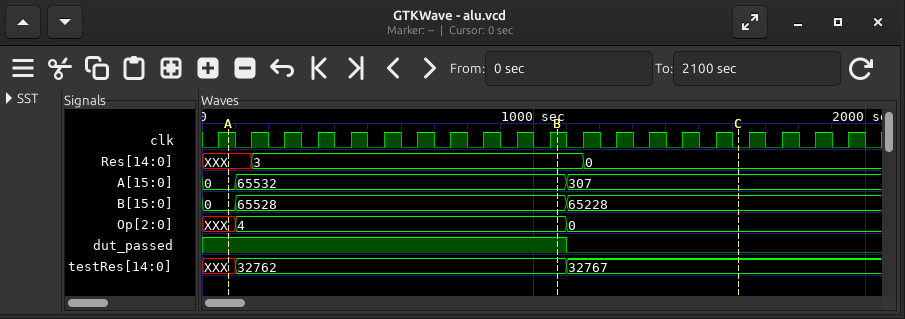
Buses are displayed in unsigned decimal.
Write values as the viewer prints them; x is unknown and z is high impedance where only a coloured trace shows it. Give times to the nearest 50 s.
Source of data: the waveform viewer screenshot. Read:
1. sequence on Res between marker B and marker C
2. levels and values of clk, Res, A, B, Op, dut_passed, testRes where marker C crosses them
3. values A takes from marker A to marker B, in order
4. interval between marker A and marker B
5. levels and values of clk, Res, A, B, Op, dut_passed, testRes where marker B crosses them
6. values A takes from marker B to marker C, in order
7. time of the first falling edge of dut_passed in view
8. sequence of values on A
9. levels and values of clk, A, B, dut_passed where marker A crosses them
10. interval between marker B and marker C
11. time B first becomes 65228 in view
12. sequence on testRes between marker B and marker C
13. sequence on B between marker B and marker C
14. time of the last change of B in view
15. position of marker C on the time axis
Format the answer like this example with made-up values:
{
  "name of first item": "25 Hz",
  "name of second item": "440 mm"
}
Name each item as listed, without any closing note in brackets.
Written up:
{
  "sequence on Res between marker B and marker C": "3, 0",
  "levels and values of clk, Res, A, B, Op, dut_passed, testRes where marker C crosses them": "clk=0, Res=0, A=307, B=65228, Op=0, dut_passed=0, testRes=32767",
  "values A takes from marker A to marker B, in order": "0, 65532",
  "interval between marker A and marker B": "1000 s",
  "levels and values of clk, Res, A, B, Op, dut_passed, testRes where marker B crosses them": "clk=1, Res=3, A=65532, B=65528, Op=4, dut_passed=1, testRes=32762",
  "values A takes from marker B to marker C, in order": "65532, 307",
  "time of the first falling edge of dut_passed in view": "1100 s",
  "sequence of values on A": "0, 65532, 307",
  "levels and values of clk, A, B, dut_passed where marker A crosses them": "clk=1, A=0, B=0, dut_passed=1",
  "interval between marker B and marker C": "550 s",
  "time B first becomes 65228 in view": "1100 s",
  "sequence on testRes between marker B and marker C": "32762, 32767",
  "sequence on B between marker B and marker C": "65528, 65228",
  "time of the last change of B in view": "1100 s",
  "position of marker C on the time axis": "1600 s"
}
